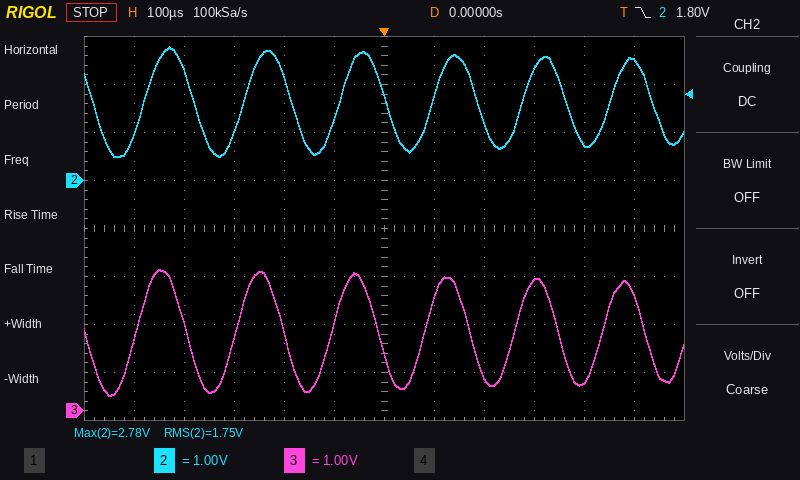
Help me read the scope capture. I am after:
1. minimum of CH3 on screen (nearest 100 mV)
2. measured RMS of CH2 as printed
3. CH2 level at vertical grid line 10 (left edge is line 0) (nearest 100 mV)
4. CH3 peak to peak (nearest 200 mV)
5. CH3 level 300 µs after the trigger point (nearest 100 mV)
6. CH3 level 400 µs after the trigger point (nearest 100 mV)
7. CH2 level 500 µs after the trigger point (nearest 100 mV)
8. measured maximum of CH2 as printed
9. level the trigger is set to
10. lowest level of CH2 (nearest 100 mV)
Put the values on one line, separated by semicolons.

300 mV; 1.75 V; 800 mV; 2.6 V; 2.7 V; 600 mV; 2.5 V; 2.78 V; 1.80 V; 500 mV
